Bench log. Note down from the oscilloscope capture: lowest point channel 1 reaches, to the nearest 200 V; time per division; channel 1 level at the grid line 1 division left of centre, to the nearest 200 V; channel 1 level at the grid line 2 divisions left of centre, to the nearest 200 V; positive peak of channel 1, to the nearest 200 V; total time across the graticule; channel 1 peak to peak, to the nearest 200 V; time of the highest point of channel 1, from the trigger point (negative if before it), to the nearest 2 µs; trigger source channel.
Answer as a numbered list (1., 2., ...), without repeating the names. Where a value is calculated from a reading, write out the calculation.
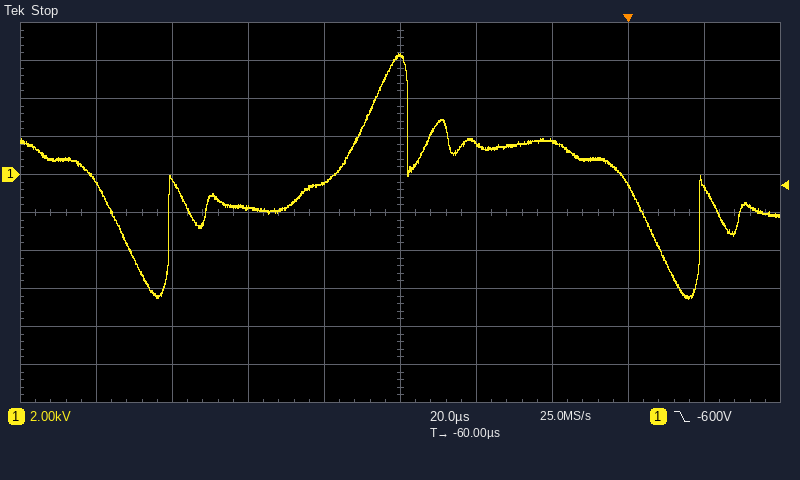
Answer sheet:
1. -6.6 kV
2. 20 µs
3. -400 V
4. -1.8 kV
5. 6.4 kV
6. 200 µs
7. 6.4 kV − (-6.6 kV) = 13.0 kV
8. -60 µs
9. channel 1
